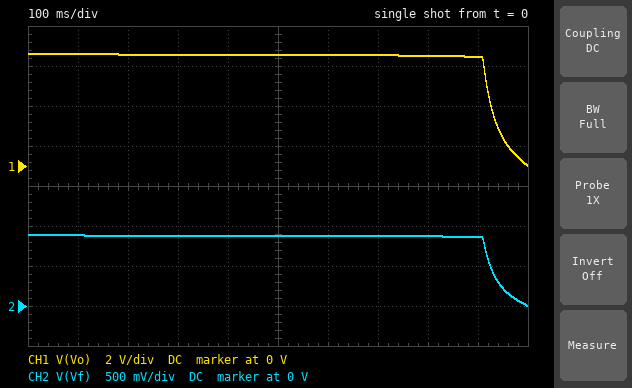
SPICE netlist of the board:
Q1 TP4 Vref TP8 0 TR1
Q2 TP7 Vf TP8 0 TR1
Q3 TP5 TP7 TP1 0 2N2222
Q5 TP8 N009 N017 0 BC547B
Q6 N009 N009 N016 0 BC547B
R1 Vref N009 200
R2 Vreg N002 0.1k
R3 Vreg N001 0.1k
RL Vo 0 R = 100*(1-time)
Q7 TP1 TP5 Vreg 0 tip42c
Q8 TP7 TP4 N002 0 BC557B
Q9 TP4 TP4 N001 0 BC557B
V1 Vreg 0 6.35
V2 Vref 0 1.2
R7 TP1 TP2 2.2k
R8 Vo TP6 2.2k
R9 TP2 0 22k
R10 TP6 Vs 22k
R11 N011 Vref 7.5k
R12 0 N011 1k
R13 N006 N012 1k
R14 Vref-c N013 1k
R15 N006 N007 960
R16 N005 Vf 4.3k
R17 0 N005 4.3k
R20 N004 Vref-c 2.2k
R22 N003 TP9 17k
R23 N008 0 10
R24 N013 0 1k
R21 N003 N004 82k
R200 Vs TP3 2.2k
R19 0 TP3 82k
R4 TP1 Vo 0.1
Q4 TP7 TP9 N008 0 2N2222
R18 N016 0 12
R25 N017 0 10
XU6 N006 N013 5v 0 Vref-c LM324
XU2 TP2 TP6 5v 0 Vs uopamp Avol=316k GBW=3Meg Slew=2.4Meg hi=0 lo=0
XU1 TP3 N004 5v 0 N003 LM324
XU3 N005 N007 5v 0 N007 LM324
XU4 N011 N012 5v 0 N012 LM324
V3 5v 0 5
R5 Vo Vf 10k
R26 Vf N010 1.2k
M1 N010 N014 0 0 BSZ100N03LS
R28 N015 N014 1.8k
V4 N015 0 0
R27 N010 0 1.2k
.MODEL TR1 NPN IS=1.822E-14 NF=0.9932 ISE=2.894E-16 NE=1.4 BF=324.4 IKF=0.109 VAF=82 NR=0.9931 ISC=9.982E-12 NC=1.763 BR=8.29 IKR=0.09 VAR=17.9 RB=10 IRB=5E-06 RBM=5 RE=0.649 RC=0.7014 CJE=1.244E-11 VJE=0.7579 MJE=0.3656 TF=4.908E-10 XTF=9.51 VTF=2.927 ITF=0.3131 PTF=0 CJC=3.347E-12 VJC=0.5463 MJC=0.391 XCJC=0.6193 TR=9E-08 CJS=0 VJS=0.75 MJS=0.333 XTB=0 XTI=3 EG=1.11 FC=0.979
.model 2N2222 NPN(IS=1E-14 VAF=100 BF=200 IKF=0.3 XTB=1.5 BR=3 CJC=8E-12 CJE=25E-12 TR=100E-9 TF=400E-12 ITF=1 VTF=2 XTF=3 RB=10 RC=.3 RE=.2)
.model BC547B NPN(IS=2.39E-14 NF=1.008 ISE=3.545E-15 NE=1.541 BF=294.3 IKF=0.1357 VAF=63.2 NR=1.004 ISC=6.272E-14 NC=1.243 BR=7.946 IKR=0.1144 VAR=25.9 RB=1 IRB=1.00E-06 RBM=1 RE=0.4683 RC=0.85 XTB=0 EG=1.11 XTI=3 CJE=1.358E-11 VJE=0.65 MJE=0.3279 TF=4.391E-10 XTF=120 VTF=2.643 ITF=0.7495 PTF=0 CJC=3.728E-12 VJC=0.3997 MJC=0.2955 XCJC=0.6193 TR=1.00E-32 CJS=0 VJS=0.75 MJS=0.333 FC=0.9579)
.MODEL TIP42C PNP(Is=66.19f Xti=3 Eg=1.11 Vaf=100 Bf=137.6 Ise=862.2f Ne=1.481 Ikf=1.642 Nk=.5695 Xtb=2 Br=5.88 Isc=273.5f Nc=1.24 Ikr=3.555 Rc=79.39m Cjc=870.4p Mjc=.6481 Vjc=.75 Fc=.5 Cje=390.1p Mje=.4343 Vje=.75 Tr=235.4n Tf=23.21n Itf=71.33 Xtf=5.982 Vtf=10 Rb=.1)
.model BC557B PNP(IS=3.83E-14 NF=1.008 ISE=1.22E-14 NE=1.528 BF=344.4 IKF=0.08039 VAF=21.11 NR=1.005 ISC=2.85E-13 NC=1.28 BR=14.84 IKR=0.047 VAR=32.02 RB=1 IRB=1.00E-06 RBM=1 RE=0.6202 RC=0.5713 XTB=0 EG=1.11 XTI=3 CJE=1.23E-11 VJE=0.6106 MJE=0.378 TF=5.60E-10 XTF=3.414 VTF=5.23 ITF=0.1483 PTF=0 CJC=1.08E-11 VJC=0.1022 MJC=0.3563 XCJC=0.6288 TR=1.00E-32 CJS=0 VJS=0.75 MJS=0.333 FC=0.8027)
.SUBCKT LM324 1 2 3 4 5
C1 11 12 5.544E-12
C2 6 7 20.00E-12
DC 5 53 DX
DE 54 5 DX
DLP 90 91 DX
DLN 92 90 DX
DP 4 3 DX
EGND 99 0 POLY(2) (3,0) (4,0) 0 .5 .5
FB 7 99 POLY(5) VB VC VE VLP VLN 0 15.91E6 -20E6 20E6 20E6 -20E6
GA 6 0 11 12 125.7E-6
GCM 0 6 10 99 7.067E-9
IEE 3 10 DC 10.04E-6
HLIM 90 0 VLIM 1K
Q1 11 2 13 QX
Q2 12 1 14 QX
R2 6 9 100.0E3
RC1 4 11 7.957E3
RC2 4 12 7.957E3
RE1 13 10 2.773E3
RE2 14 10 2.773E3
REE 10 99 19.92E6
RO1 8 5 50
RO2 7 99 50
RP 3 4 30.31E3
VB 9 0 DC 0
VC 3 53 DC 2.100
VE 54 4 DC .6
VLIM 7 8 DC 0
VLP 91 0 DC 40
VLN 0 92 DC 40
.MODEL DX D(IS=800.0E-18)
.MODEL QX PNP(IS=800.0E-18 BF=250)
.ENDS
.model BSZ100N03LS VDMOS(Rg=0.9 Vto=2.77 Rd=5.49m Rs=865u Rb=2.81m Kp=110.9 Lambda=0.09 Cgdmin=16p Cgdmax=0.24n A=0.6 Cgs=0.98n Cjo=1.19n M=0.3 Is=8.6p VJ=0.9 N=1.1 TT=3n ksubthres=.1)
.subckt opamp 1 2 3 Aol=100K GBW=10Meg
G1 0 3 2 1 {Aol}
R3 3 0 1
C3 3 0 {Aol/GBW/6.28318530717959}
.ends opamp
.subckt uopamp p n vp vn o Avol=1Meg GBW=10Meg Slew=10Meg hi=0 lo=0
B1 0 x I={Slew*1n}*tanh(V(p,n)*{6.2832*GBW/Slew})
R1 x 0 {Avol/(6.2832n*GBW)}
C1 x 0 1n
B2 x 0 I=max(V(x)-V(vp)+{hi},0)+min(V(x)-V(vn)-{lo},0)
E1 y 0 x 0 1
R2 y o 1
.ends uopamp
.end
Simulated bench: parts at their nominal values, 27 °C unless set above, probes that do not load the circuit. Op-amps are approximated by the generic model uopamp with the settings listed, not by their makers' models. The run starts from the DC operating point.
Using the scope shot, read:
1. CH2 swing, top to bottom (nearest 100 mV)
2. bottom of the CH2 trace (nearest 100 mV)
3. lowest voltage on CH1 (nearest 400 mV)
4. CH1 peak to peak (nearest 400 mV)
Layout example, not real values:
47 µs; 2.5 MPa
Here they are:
900 mV; 0 V; 0 V; 5.6 V
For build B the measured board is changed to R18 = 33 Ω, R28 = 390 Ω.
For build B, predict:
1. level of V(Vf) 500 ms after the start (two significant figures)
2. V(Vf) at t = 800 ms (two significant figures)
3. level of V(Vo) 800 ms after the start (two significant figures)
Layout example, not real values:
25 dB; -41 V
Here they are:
860 mV; 850 mV; 5.4 V
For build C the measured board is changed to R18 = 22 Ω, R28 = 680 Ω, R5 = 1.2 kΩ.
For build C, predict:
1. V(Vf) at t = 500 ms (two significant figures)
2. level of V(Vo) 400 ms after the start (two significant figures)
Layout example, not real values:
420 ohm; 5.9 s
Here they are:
1.2 V; 2.0 V
